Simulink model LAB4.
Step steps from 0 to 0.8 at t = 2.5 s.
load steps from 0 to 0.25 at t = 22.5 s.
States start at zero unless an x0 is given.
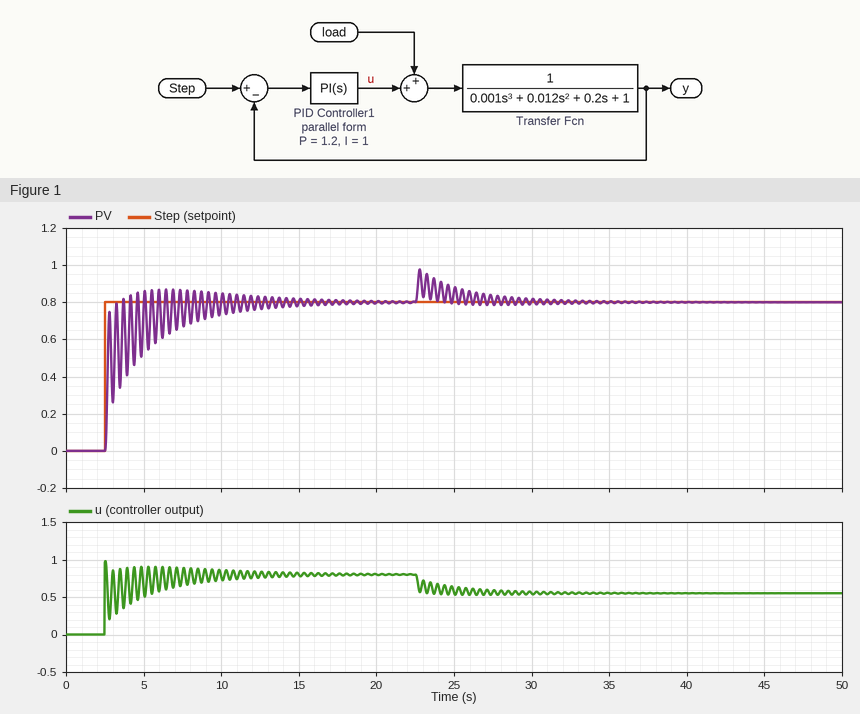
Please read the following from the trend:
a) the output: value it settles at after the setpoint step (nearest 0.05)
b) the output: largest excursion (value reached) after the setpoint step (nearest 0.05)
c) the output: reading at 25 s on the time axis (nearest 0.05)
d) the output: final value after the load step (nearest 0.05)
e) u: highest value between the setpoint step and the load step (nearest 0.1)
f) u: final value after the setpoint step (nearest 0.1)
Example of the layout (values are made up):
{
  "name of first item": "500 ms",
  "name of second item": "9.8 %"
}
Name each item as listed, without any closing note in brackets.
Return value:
{
  "the output: value it settles at after the setpoint step": "0.80",
  "the output: largest excursion (value reached) after the setpoint step": "0.85",
  "the output: reading at 25 s on the time axis": "0.85",
  "the output: final value after the load step": "0.80",
  "u: highest value between the setpoint step and the load step": "1.0",
  "u: final value after the setpoint step": "0.8"
}
